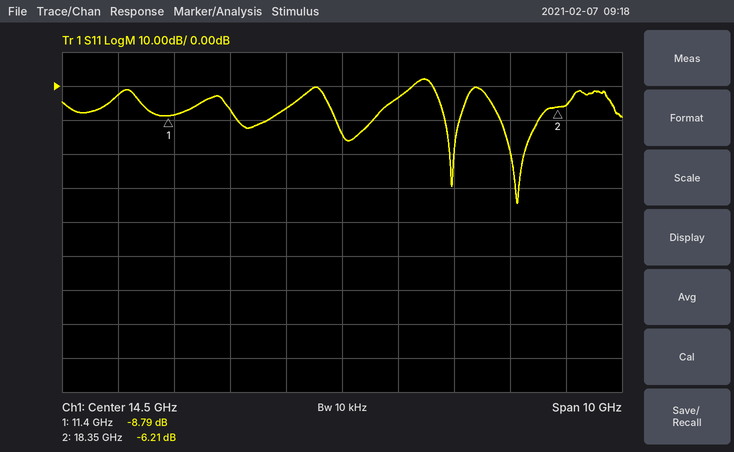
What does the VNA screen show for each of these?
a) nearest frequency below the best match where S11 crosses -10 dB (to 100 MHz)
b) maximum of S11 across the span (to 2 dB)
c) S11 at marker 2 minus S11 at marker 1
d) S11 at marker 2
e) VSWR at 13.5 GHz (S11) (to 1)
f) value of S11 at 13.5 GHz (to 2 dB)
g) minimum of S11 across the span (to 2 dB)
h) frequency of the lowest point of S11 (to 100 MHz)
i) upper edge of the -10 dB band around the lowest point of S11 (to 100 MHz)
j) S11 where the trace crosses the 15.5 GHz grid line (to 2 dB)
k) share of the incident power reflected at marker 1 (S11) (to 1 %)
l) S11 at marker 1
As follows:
17.3 GHz
2 dB
2.58 dB
-6.21 dB
3
-6 dB
-34 dB
17.6 GHz
18.0 GHz
-4 dB
13 %
-8.79 dB
